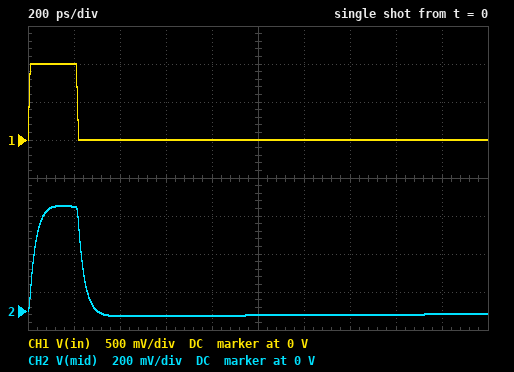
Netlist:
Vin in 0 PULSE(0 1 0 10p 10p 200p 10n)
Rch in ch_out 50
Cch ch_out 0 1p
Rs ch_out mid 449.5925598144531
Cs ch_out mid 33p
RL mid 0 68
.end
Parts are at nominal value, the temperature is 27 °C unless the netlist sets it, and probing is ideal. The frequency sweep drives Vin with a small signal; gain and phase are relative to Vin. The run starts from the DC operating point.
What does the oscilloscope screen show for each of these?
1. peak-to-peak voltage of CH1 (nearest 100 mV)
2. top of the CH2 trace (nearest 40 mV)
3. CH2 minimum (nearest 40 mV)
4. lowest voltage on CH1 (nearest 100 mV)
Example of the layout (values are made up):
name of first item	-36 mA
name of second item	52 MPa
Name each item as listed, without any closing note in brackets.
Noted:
peak-to-peak voltage of CH1	1.0 V
top of the CH2 trace	560 mV
CH2 minimum	-40 mV
lowest voltage on CH1	0 V
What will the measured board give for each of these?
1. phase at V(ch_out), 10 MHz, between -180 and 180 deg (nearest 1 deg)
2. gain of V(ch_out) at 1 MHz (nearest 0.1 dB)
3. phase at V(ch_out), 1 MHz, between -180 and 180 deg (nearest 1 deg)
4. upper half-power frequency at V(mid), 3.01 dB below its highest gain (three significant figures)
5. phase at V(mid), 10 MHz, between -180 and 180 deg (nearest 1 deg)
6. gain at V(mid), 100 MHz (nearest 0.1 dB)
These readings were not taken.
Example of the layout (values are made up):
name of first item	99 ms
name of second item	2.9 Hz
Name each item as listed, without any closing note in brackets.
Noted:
phase at V(ch_out), 10 MHz, between -180 and 180 deg	-4 deg
gain of V(ch_out) at 1 MHz	-0.8 dB
phase at V(ch_out), 1 MHz, between -180 and 180 deg	0 deg
upper half-power frequency at V(mid), 3.01 dB below its highest gain	5.65 GHz
phase at V(mid), 10 MHz, between -180 and 180 deg	32 deg
gain at V(mid), 100 MHz	-5.8 dB
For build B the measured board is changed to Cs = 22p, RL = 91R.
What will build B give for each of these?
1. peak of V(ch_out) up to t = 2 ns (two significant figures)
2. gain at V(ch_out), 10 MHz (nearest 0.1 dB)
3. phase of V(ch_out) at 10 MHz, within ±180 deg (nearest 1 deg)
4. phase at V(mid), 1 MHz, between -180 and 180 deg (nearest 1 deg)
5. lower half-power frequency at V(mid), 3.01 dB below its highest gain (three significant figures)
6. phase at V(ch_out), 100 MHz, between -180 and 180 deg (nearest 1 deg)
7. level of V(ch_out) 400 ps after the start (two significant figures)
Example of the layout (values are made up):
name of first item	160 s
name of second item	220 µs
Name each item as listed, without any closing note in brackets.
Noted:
peak of V(ch_out) up to t = 2 ns	660 mV
gain at V(ch_out), 10 MHz	-0.8 dB
phase of V(ch_out) at 10 MHz, within ±180 deg	-3 deg
phase at V(mid), 1 MHz, between -180 and 180 deg	3 deg
lower half-power frequency at V(mid), 3.01 dB below its highest gain	61.3 MHz
phase at V(ch_out), 100 MHz, between -180 and 180 deg	-11 deg
level of V(ch_out) 400 ps after the start	24 mV
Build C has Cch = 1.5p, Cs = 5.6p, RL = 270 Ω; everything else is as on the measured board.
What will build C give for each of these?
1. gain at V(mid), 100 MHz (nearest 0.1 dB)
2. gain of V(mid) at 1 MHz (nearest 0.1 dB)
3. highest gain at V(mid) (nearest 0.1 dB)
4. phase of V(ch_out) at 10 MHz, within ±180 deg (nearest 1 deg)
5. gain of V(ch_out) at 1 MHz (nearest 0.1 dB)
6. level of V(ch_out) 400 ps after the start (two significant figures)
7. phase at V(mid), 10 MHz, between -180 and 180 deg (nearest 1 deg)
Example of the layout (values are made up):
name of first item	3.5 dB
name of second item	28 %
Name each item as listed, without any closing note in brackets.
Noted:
gain at V(mid), 100 MHz	-5.2 dB
gain of V(mid) at 1 MHz	-9.1 dB
highest gain at V(mid)	-2.0 dB
phase of V(ch_out) at 10 MHz, within ±180 deg	-1 deg
gain of V(ch_out) at 1 MHz	-0.6 dB
level of V(ch_out) 400 ps after the start	58 mV
phase at V(mid), 10 MHz, between -180 and 180 deg	5 deg
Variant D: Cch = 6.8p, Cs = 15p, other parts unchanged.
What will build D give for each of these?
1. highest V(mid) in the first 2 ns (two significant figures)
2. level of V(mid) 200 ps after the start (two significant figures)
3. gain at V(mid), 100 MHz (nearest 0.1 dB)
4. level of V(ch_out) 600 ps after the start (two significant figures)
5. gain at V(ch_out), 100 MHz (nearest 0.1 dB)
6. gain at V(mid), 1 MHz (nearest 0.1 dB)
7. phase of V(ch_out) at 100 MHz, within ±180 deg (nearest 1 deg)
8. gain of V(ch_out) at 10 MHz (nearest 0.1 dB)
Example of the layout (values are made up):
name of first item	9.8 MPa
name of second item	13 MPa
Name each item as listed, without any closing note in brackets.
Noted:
highest V(mid) in the first 2 ns	340 mV
level of V(mid) 200 ps after the start	330 mV
gain at V(mid), 100 MHz	-8.6 dB
level of V(ch_out) 600 ps after the start	82 mV
gain at V(ch_out), 100 MHz	-2.5 dB
gain at V(mid), 1 MHz	-18.4 dB
phase of V(ch_out) at 100 MHz, within ±180 deg	-21 deg
gain of V(ch_out) at 10 MHz	-0.8 dB
